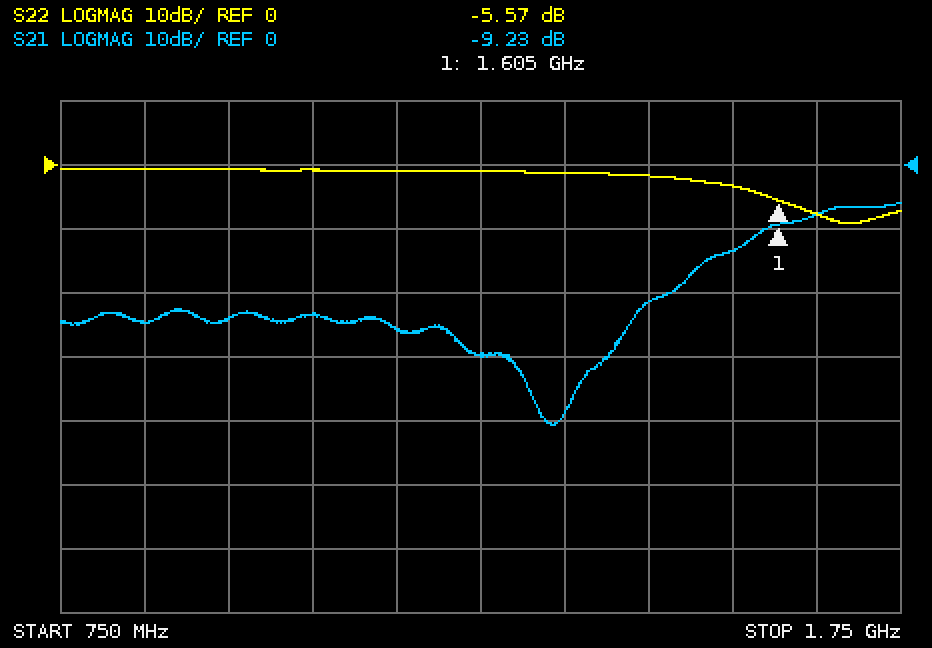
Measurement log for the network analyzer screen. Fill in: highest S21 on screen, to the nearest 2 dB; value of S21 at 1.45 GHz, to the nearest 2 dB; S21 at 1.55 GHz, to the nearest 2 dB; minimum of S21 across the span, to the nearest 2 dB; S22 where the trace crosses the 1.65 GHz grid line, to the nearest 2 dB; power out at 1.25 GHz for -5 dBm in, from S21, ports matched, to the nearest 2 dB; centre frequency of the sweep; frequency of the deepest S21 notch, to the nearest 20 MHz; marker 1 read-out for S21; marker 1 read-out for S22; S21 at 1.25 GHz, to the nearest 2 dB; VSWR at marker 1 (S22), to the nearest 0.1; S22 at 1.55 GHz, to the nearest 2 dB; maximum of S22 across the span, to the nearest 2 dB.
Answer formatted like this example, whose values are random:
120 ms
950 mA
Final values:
-6 dB
-22 dB
-14 dB
-40 dB
-8 dB
-34 dBm
1.25 GHz
1.34 GHz
-9.23 dB
-5.57 dB
-30 dB
3.2
-4 dB
0 dB
